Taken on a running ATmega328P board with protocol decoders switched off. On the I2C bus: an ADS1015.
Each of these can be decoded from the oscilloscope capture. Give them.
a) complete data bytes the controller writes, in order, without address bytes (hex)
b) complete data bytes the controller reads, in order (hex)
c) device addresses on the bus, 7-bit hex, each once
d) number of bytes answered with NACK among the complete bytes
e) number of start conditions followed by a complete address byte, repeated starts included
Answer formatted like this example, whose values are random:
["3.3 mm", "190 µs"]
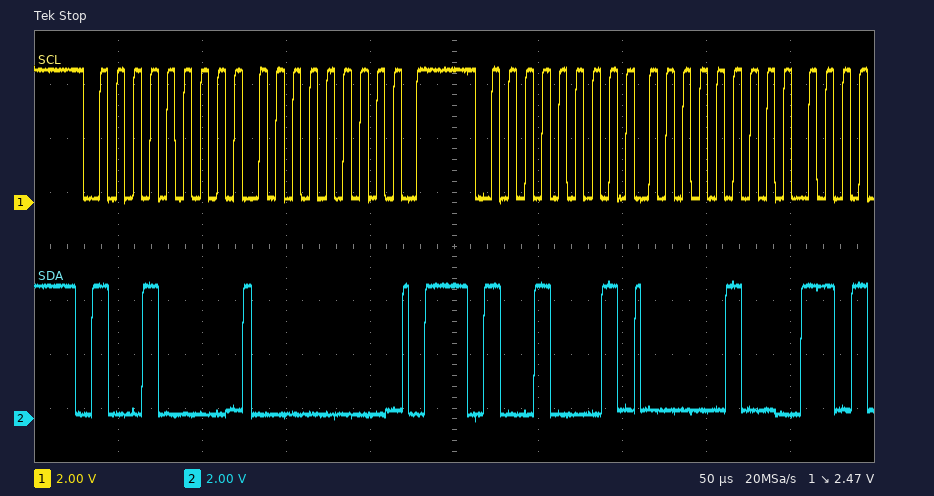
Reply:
["00", "04", "0x48", "0", "2"]
